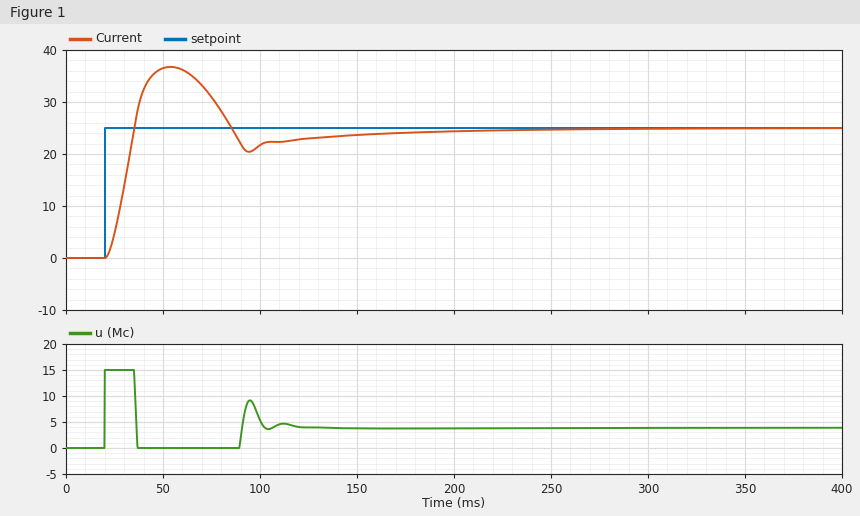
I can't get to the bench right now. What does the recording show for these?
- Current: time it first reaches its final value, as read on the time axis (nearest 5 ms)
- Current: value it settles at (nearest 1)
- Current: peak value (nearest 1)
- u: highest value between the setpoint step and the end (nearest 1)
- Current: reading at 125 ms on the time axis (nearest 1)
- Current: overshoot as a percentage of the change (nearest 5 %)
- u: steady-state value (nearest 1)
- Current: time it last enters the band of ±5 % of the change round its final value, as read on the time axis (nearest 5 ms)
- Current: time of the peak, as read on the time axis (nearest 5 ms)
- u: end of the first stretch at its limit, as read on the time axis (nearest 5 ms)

35 ms
25
37
15
23
45 %
4
155 ms
55 ms
35 ms
